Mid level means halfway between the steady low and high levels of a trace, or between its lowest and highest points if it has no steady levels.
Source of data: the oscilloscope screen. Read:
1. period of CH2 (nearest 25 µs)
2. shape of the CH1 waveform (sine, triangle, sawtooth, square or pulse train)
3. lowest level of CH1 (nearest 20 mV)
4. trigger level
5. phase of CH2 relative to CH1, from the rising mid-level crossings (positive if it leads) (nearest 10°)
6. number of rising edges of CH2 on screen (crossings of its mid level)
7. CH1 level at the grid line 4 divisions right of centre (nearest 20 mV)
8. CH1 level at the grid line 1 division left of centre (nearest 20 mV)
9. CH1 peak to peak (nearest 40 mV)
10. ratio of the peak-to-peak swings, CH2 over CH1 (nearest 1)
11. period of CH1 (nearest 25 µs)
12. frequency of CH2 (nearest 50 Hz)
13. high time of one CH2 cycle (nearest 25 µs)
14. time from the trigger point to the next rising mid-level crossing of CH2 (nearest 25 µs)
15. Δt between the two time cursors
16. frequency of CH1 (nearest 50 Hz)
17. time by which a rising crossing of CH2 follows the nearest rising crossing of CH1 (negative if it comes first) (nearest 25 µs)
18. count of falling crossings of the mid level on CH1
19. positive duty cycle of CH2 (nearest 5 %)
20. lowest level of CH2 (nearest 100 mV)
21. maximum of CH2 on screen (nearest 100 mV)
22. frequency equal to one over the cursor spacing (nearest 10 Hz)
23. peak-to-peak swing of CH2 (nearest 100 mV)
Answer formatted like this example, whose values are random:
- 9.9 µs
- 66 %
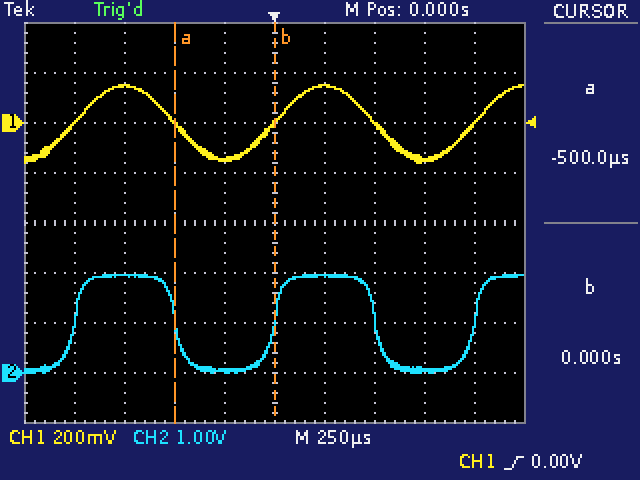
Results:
- 1.000 ms
- sine
- -160 mV
- 0.00 V
- 0°
- 3
- 0 mV
- -140 mV
- 320 mV
- 6
- 1.000 ms
- 1.00 kHz
- 500 µs
- 1.000 ms
- 500 µs
- 1.00 kHz
- 0 µs
- 2
- 50 %
- 0.0 V
- 2.0 V
- 2.00 kHz
- 2.0 V
